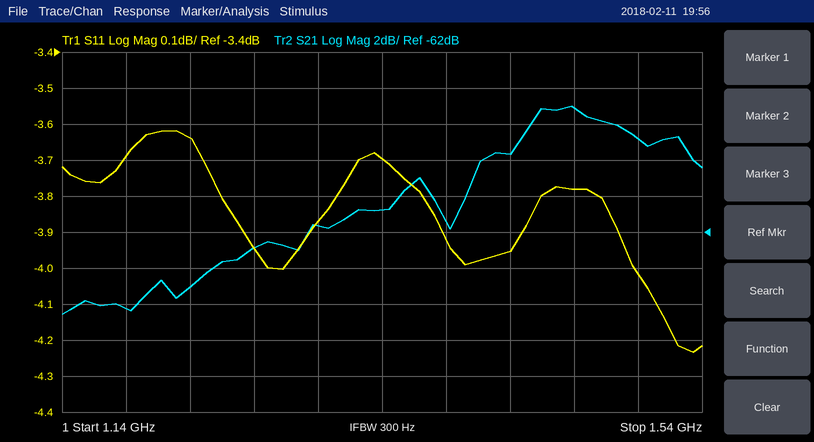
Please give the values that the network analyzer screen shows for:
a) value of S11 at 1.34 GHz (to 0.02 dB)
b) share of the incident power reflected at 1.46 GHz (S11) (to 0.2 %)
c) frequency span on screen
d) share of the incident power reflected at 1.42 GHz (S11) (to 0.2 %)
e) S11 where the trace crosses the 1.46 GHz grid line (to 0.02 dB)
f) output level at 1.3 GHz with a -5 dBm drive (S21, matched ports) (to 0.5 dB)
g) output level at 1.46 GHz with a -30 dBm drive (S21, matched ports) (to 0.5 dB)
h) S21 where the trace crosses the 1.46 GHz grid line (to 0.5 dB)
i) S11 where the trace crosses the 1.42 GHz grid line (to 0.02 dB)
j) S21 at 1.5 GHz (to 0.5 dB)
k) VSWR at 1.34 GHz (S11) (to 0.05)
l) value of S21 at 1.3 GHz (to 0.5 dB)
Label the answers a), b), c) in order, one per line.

a) -3.70 dB
b) 41.8 %
c) 400 MHz
d) 40.2 %
e) -3.78 dB
f) -66.5 dBm
g) -85.0 dBm
h) -55.0 dB
i) -3.96 dB
j) -57.0 dB
k) 4.75
l) -61.5 dB
